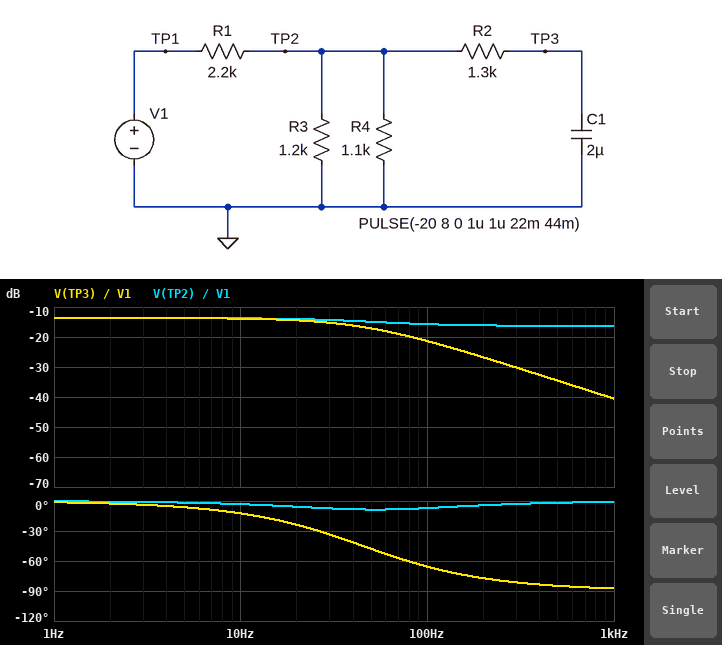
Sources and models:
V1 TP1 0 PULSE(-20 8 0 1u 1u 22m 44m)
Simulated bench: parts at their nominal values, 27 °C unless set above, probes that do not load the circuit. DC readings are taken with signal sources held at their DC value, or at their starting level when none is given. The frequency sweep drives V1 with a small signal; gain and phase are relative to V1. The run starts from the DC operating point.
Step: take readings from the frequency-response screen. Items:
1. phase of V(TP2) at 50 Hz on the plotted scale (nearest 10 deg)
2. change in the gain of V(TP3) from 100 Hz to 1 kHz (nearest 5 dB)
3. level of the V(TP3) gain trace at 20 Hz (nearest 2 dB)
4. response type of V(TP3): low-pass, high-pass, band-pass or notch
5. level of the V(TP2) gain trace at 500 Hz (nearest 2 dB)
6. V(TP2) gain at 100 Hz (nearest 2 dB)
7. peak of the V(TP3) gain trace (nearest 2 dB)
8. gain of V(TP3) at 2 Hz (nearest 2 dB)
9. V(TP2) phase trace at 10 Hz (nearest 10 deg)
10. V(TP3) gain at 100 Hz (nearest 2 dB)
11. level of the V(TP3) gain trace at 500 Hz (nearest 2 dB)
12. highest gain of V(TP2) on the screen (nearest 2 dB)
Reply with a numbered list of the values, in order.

1. -10 deg
2. -20 dB
3. -14 dB
4. low-pass
5. -16 dB
6. -16 dB
7. -14 dB
8. -14 dB
9. 0 deg
10. -22 dB
11. -34 dB
12. -14 dB
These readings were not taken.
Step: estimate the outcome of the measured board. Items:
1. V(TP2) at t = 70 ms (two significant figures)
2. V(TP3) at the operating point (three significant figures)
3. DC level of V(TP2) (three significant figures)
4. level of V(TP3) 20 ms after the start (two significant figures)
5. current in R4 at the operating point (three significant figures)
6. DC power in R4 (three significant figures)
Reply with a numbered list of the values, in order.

1. -3.7 V
2. -4.14 V
3. -4.14 V
4. 1.6 V
5. 3.76 mA
6. 15.6 mW
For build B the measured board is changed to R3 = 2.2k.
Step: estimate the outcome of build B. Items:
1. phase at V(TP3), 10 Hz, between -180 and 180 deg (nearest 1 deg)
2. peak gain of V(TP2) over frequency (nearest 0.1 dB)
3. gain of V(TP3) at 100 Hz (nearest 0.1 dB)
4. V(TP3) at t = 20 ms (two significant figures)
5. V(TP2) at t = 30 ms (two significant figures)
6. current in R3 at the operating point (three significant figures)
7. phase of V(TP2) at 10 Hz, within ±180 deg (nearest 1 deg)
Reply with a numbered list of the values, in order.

1. -13 deg
2. -12.0 dB
3. -20.1 dB
4. 2.0 V
5. -4.8 V
6. 2.27 mA
7. -4 deg
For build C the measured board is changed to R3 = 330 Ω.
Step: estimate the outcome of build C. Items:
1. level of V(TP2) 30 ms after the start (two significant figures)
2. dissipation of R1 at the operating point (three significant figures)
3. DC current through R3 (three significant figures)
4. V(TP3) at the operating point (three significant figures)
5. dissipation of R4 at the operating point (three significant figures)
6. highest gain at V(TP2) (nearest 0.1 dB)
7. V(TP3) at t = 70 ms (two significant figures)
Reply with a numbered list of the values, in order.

1. -2.0 V
2. 146 mW
3. 6.27 mA
4. -2.07 V
5. 3.89 mW
6. -19.7 dB
7. -1.3 V
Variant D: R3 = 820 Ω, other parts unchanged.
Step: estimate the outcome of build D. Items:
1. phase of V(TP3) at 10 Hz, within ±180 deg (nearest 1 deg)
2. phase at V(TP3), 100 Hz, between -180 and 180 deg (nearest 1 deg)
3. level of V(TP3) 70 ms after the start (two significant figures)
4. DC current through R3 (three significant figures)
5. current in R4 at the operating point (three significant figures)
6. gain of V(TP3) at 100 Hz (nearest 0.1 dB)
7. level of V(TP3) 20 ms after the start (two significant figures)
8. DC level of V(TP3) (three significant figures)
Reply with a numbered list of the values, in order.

1. -12 deg
2. -65 deg
3. -2.0 V
4. 4.29 mA
5. 3.20 mA
6. -22.5 dB
7. 1.4 V
8. -3.52 V
